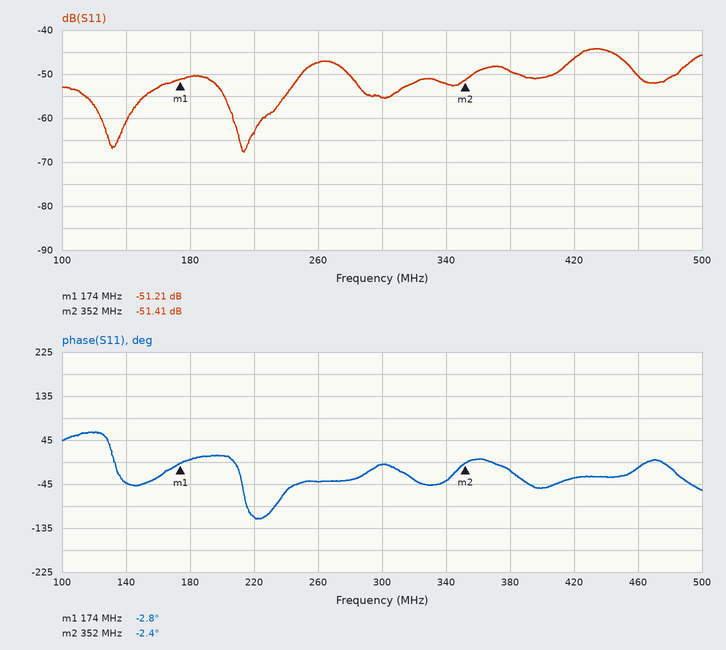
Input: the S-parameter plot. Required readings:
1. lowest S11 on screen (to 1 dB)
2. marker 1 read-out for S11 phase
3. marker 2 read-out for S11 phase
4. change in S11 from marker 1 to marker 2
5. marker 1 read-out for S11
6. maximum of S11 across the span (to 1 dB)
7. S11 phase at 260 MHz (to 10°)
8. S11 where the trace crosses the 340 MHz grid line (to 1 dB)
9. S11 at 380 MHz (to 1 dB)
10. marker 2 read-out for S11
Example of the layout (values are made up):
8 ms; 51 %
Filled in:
-68 dB; -2.8°; -2.4°; -0.20 dB; -51.21 dB; -44 dB; -40°; -52 dB; -49 dB; -51.41 dB
